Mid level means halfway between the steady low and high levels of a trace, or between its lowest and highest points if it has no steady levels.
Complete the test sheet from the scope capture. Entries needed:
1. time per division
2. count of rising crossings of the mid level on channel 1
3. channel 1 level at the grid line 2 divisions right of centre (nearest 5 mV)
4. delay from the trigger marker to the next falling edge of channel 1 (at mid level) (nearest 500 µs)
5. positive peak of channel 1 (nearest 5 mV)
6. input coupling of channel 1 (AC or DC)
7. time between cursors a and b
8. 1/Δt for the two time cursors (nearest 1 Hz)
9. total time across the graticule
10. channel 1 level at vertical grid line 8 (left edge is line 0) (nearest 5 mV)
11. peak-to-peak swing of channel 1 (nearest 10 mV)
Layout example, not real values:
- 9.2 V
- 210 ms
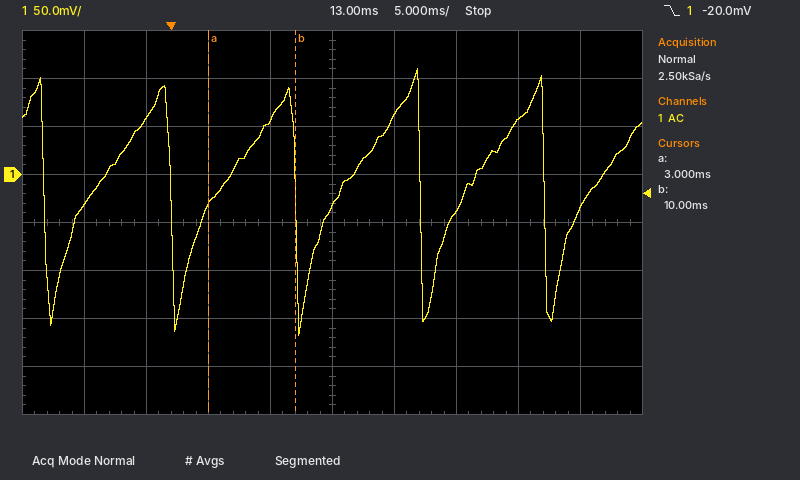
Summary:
- 5 ms
- 5
- -40 mV
- 10.0 ms
- 110 mV
- AC
- 7.0 ms
- 143 Hz
- 50 ms
- 55 mV
- 280 mV
